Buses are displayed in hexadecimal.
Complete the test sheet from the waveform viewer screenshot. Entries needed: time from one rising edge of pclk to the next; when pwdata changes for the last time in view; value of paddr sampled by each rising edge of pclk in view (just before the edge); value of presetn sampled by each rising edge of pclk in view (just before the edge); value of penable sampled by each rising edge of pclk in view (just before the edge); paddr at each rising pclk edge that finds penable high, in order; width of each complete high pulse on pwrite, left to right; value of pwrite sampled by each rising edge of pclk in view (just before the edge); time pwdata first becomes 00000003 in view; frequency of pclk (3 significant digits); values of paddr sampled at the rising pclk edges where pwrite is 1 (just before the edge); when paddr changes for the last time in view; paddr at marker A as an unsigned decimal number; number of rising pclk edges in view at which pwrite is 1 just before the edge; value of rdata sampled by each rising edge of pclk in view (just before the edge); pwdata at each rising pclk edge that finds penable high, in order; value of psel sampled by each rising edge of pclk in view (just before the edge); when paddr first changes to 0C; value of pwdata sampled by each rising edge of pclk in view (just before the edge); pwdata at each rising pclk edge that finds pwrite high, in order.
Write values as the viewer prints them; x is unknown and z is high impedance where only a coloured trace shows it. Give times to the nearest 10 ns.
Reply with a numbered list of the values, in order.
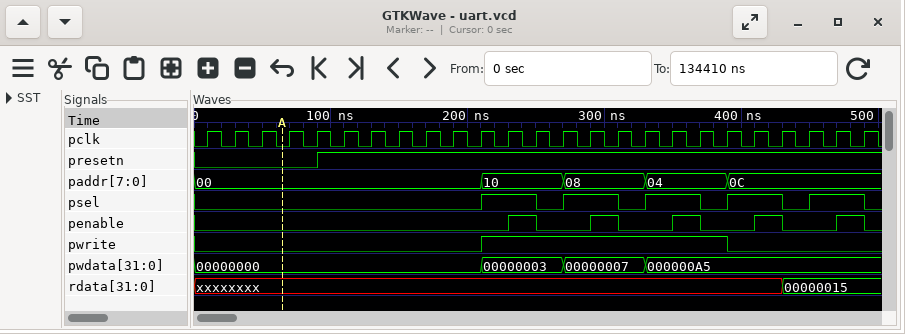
1. 20 ns
2. 330 ns
3. 00, 00, 00, 00, 00, 00, 00, 00, 00, 00, 00, 10, 10, 10, 08, 08, 08, 04, 04, 04, 0C, 0C, 0C, 0C, 0C
4. 0 0 0 0 0 1 1 1 1 1 1 1 1 1 1 1 1 1 1 1 1 1 1 1 1
5. 0 0 0 0 0 0 0 0 0 0 0 0 1 0 0 1 0 0 1 0 0 1 0 0 1
6. 10, 08, 04, 0C, 0C
7. 180 ns
8. 0 0 0 0 0 0 0 0 0 0 0 1 1 1 1 1 1 1 1 1 0 0 0 0 0
9. 210 ns
10. 50.0 MHz
11. 10, 10, 10, 08, 08, 08, 04, 04, 04
12. 390 ns
13. 0
14. 9
15. xxxxxxxx, xxxxxxxx, xxxxxxxx, xxxxxxxx, xxxxxxxx, xxxxxxxx, xxxxxxxx, xxxxxxxx, xxxxxxxx, xxxxxxxx, xxxxxxxx, xxxxxxxx, xxxxxxxx, xxxxxxxx, xxxxxxxx, xxxxxxxx, xxxxxxxx, xxxxxxxx, xxxxxxxx, xxxxxxxx, xxxxxxxx, xxxxxxxx, 00000015, 00000015, 00000015
16. 00000003, 00000007, 000000A5, 000000A5, 000000A5
17. 0 0 0 0 0 0 0 0 0 0 0 1 1 0 1 1 0 1 1 0 1 1 0 1 1
18. 390 ns
19. 00000000, 00000000, 00000000, 00000000, 00000000, 00000000, 00000000, 00000000, 00000000, 00000000, 00000000, 00000003, 00000003, 00000003, 00000007, 00000007, 00000007, 000000A5, 000000A5, 000000A5, 000000A5, 000000A5, 000000A5, 000000A5, 000000A5
20. 00000003, 00000003, 00000003, 00000007, 00000007, 00000007, 000000A5, 000000A5, 000000A5
